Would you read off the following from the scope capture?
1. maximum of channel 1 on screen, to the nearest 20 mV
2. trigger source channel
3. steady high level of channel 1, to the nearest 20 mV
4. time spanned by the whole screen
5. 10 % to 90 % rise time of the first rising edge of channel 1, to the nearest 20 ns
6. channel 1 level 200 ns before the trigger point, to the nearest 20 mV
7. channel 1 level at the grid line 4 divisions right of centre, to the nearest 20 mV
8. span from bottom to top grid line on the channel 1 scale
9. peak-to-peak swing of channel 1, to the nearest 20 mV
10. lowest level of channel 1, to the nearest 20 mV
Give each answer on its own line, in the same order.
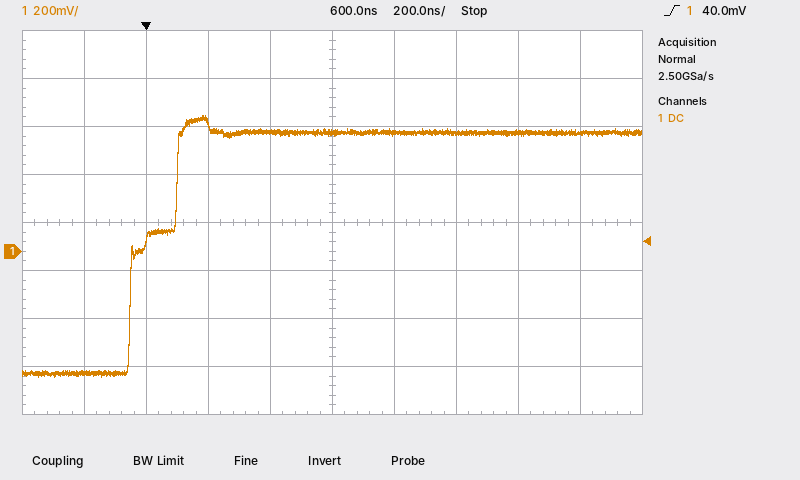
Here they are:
560 mV
channel 1
500 mV
2 µs
160 ns
-500 mV
500 mV
1.6 V
1.08 V
-520 mV
